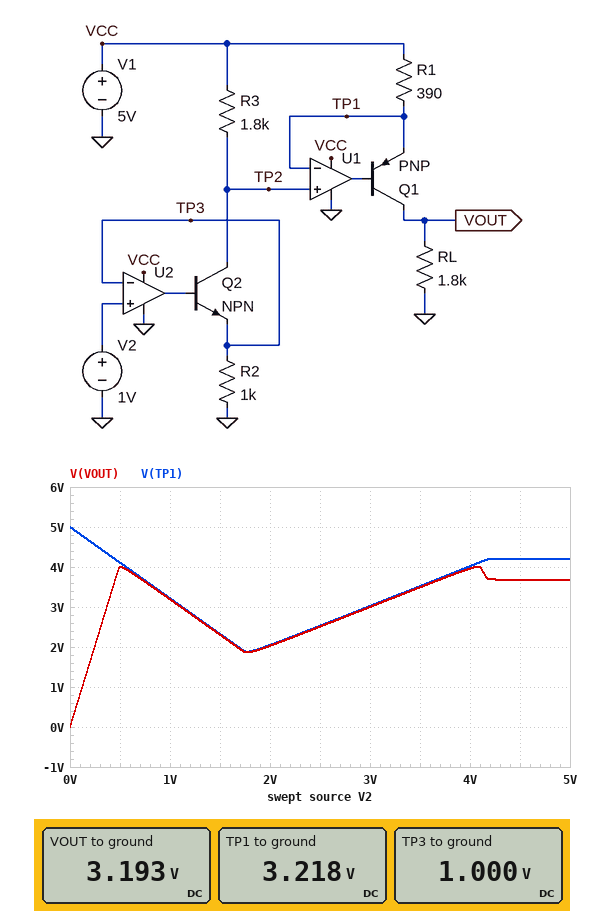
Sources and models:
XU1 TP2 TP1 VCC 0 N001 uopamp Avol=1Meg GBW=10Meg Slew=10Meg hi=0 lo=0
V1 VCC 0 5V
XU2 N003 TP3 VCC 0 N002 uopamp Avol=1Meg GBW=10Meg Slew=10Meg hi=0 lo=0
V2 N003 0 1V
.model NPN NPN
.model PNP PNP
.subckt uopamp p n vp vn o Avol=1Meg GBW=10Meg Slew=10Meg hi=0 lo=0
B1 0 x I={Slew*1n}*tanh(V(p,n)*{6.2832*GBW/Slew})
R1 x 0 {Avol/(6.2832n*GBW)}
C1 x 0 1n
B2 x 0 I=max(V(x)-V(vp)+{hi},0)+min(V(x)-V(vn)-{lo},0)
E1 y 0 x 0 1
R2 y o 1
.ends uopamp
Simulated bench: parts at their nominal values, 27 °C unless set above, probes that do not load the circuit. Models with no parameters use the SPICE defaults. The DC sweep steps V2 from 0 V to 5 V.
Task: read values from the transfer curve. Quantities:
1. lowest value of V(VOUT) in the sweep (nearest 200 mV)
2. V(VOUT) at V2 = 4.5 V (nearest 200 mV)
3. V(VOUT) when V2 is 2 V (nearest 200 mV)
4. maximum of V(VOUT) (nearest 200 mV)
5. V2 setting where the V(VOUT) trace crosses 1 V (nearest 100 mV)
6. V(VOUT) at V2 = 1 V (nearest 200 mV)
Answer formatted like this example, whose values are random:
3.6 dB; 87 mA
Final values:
0 V; 3.6 V; 2.0 V; 4.0 V; 100 mV; 3.2 V
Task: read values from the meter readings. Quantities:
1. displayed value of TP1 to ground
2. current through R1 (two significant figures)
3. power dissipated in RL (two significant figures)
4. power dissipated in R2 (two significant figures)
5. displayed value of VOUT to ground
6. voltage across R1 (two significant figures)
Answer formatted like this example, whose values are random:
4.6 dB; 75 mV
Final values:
3.218 V; 4.6 mA; 5.7 mW; 1.0 mW; 3.193 V; 1.8 V
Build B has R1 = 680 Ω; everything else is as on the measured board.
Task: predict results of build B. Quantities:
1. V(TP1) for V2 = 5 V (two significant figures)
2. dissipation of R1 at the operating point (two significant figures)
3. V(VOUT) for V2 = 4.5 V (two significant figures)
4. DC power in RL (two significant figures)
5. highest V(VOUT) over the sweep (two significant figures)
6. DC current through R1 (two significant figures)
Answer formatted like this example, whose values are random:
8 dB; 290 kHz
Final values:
4.2 V; 4.7 mW; 2.1 V; 5.6 mW; 3.5 V; 2.6 mA
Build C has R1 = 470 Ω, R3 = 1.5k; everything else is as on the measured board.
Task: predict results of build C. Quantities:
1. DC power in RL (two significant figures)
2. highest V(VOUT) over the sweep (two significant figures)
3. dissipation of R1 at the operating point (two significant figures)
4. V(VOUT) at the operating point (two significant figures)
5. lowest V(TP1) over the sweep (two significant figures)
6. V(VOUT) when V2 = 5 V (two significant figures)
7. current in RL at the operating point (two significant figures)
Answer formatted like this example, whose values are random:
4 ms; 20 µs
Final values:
6.7 mW; 3.9 V; 4.7 mW; 3.5 V; 2.1 V; 3.0 V; 1.9 mA
